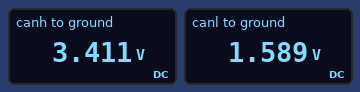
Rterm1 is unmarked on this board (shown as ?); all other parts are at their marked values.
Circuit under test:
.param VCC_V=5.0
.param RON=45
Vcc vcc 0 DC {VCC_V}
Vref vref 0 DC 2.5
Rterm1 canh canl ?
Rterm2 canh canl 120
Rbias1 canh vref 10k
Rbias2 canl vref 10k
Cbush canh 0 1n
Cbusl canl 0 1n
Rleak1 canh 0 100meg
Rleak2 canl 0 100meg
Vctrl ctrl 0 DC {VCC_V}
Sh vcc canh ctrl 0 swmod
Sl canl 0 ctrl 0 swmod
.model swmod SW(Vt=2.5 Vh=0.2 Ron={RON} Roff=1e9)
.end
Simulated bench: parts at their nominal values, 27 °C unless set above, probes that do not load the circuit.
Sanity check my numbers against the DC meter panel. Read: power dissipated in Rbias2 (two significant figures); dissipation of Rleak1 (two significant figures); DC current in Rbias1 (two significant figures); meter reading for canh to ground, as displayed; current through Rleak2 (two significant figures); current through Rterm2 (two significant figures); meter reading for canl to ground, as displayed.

83 µW
120 nW
91 µA
3.411 V
16 nA
15 mA
1.589 V
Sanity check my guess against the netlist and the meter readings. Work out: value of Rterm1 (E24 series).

91 Ω
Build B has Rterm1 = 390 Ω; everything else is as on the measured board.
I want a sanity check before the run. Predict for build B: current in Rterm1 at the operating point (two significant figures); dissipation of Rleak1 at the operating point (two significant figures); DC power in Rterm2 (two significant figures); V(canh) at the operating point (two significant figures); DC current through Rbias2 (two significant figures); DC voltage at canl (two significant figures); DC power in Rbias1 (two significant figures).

6.5 mA
140 nW
53 mW
3.8 V
130 µA
1.2 V
160 µW
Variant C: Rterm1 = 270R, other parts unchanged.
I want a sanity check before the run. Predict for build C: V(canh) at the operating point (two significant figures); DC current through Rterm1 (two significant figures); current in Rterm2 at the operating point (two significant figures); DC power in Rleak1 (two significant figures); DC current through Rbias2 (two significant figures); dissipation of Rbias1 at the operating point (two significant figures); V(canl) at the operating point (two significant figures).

3.7 V
8.9 mA
20 mA
140 nW
120 µA
140 µW
1.3 V
